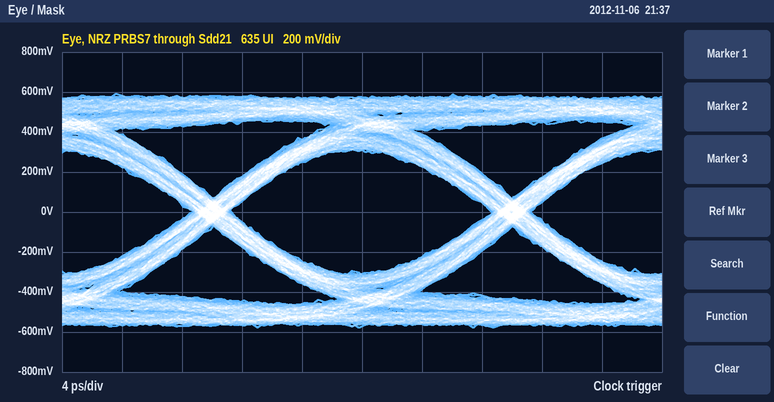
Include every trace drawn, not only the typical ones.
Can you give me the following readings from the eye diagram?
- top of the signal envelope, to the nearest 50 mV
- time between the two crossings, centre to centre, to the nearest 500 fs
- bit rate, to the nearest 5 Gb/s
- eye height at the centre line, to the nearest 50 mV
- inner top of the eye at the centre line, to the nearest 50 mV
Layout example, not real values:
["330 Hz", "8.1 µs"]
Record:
["600 mV", "20.0 ps", "50 Gb/s", "600 mV", "300 mV"]
